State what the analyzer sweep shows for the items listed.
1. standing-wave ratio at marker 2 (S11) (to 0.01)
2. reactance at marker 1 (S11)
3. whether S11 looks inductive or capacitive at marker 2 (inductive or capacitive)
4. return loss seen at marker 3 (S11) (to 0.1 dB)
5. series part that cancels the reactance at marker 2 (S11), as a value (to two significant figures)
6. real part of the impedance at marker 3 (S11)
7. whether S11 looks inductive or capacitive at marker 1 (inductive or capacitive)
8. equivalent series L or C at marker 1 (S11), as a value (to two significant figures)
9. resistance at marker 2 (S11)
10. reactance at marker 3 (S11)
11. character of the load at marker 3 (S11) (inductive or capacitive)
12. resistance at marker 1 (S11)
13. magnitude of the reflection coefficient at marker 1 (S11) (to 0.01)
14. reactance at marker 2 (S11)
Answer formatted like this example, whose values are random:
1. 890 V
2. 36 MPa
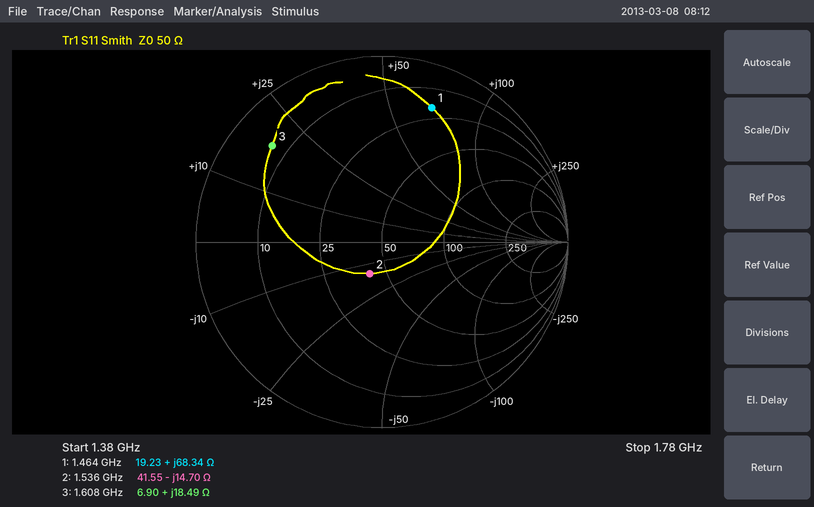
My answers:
1. 1.45
2. +68.34 Ω
3. capacitive
4. 2.1 dB
5. 1.5 nH
6. 6.90 Ω
7. inductive
8. 7.4 nH
9. 41.55 Ω
10. +18.49 Ω
11. inductive
12. 19.23 Ω
13. 0.77
14. -14.70 Ω
